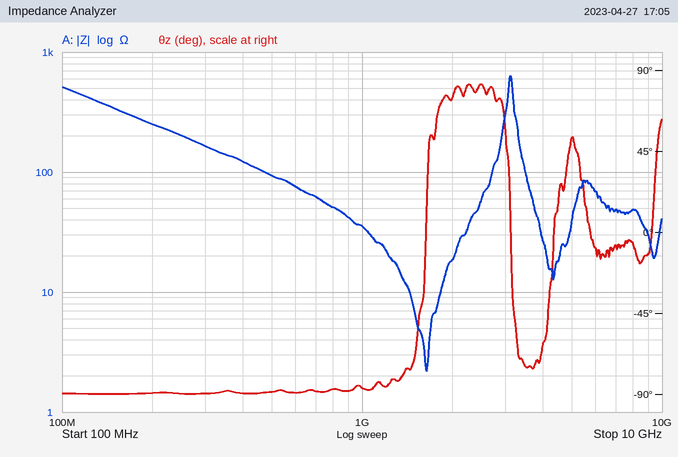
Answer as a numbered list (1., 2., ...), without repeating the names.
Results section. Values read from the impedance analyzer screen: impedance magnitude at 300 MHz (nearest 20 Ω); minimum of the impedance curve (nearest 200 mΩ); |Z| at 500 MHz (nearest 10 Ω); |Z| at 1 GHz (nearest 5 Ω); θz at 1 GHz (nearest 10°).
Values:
1. 160 Ω
2. 2.2 Ω
3. 90 Ω
4. 35 Ω
5. -90°
